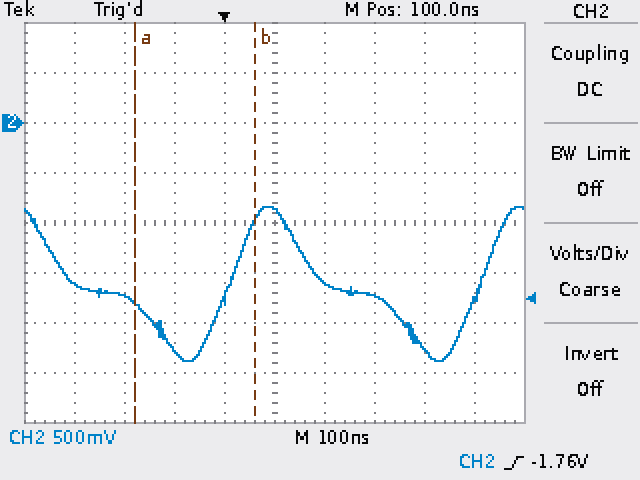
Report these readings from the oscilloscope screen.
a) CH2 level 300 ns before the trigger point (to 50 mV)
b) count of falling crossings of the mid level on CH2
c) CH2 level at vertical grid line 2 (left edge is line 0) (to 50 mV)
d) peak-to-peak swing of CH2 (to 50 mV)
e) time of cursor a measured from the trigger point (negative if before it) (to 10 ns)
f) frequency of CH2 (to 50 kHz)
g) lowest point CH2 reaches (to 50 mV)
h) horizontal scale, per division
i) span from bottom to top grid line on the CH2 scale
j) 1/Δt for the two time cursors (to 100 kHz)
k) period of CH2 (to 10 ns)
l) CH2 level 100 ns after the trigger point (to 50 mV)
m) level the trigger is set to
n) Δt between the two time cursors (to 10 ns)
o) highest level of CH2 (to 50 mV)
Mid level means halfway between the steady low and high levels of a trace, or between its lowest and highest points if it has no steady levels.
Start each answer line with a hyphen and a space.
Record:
- -1.60 V
- 2
- -1.75 V
- 1.55 V
- -180 ns
- 2.00 MHz
- -2.40 V
- 100 ns
- 4 V
- 4.2 MHz
- 500 ns
- -850 mV
- -1.76 V
- 240 ns
- -850 mV
